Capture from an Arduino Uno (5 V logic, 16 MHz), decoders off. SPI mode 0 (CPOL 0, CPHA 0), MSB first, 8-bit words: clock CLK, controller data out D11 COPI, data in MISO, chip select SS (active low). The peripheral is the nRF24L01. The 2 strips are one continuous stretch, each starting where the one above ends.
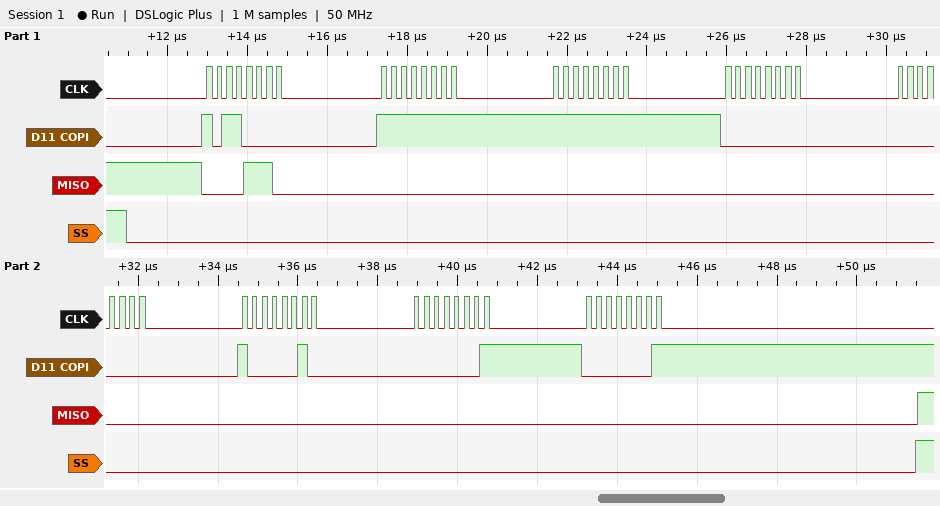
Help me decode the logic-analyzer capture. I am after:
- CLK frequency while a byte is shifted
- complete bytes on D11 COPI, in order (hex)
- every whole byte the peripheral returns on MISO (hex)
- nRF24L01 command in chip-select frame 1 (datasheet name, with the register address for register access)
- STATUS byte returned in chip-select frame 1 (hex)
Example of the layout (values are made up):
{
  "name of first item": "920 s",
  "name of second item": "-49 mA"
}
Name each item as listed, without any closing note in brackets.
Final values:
{
  "CLK frequency while a byte is shifted": "4 MHz",
  "complete bytes on D11 COPI, in order": "B0 FF FF 00 00 82 01 01",
  "every whole byte the peripheral returns on MISO": "0E 00 00 00 00 00 00 00",
  "nRF24L01 command in chip-select frame 1": "W_TX_PAYLOAD_NOACK",
  "STATUS byte returned in chip-select frame 1": "0x0E"
}
